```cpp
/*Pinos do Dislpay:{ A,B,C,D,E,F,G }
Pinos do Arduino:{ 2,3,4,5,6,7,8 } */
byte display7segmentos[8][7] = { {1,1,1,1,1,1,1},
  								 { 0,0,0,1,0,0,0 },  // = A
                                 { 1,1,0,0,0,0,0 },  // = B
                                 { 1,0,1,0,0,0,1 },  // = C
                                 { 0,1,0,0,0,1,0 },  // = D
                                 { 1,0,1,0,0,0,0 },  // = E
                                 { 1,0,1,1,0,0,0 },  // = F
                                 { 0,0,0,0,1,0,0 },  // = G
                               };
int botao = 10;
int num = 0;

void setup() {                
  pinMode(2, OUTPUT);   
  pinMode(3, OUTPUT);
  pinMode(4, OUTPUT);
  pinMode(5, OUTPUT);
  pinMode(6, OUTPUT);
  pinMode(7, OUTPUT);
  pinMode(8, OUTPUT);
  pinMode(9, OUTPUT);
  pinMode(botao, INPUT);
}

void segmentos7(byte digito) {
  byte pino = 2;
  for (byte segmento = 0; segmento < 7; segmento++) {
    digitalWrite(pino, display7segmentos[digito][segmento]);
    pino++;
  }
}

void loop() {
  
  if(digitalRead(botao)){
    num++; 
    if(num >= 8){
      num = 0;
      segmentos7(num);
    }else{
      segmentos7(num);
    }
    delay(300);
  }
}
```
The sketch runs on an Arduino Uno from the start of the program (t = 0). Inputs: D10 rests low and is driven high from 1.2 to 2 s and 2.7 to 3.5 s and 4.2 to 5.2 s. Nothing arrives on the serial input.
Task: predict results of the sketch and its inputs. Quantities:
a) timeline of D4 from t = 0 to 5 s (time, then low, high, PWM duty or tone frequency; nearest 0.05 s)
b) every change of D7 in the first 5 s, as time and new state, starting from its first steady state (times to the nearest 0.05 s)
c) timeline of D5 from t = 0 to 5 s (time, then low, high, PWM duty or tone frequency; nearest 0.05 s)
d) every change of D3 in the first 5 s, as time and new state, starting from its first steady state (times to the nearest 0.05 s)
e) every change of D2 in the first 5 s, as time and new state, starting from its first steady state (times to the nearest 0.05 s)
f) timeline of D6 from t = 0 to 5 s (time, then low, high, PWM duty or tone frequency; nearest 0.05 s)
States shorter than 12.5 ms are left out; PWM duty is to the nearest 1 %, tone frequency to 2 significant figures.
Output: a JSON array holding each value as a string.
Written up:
["0 s low; 1.8 s high; 2.7 s low; 3 s high; 4.2 s low; 4.5 s high; 4.8 s low", "0 s low; 2.7 s high; 3 s low; 4.5 s high; 4.8 s low", "0 s low; 1.2 s high; 1.5 s low; 3.3 s high; 4.2 s low; 4.5 s high", "0 s low; 1.5 s high; 1.8 s low; 2.7 s high; 3 s low; 4.5 s high; 4.8 s low", "0 s low; 1.5 s high; 2.7 s low; 3 s high; 4.2 s low; 4.5 s high; 4.8 s low", "0 s low; 4.2 s high; 4.8 s low"]
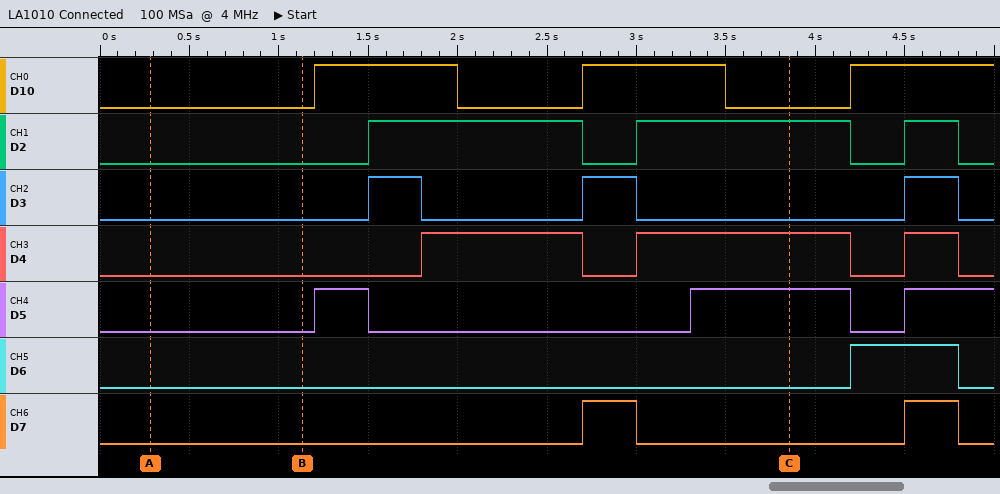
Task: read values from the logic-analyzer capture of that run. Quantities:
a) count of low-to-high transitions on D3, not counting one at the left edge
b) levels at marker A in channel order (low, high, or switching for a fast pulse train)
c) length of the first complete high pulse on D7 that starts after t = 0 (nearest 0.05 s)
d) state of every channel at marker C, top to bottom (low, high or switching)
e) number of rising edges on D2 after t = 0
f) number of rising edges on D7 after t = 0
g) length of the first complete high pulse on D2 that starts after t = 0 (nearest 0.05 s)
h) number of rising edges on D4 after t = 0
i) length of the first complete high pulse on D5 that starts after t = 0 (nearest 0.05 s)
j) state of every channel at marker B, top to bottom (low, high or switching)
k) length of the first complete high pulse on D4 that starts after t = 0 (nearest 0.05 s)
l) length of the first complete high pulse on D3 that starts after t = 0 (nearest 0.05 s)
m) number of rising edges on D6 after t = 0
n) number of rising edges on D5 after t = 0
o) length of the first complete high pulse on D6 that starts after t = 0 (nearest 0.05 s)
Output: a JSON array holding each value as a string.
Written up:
["3", "D10 low, D2 low, D3 low, D4 low, D5 low, D6 low, D7 low", "0.30 s", "D10 low, D2 high, D3 low, D4 high, D5 high, D6 low, D7 low", "3", "2", "1.20 s", "3", "0.30 s", "D10 low, D2 low, D3 low, D4 low, D5 low, D6 low, D7 low", "0.90 s", "0.30 s", "1", "3", "0.60 s"]
